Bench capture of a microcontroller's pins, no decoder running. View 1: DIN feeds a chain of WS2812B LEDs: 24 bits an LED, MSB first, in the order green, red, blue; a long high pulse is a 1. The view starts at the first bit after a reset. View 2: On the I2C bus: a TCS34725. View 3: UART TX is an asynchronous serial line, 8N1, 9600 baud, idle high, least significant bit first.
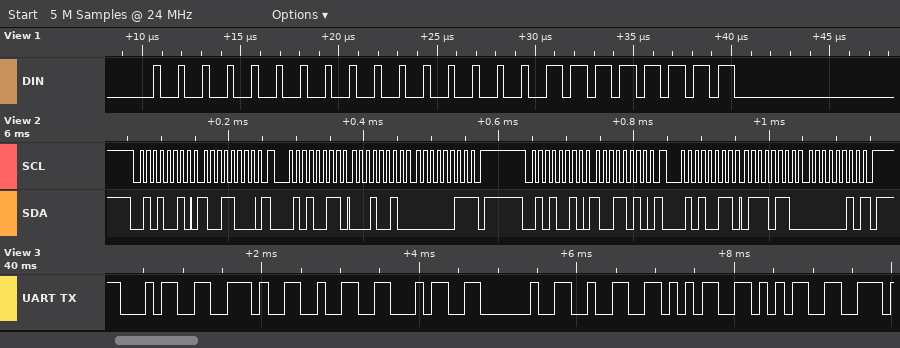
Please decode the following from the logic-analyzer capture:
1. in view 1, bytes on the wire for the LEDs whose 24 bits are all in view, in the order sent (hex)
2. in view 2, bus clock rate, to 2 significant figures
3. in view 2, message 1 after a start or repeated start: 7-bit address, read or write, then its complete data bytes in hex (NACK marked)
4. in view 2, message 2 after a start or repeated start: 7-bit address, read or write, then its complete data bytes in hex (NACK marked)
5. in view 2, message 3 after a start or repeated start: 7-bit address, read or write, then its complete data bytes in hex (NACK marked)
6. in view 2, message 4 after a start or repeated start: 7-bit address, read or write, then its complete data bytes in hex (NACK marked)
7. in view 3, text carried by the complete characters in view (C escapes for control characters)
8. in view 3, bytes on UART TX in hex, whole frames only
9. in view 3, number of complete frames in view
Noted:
00 00 FF
100 kHz
0x29 write: 98
0x29 read: 12 03 NACK
0x29 write: 9A
0x29 read: 76 02 NACK
"4.24 255"
34 2E 32 34 20 32 35 35
8
